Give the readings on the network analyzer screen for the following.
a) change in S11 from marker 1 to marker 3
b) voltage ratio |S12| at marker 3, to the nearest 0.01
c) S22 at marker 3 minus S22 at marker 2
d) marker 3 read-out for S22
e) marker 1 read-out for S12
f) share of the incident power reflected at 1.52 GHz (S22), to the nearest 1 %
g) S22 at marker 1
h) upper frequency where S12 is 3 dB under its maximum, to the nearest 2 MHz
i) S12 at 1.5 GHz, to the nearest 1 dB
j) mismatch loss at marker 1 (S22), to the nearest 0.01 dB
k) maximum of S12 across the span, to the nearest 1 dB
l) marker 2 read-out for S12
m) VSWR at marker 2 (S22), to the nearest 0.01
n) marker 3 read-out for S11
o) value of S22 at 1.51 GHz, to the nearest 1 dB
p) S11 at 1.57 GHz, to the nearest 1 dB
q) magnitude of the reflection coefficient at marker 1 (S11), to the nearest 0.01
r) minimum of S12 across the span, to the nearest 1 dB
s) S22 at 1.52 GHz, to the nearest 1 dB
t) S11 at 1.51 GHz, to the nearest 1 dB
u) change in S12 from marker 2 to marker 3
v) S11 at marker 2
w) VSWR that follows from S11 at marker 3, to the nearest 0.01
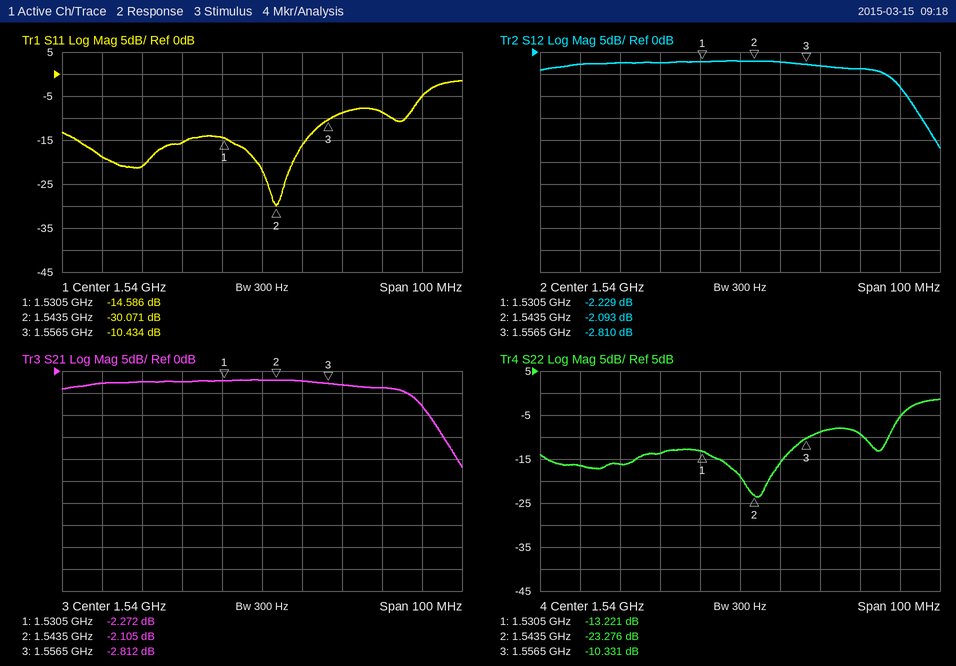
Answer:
4.152 dB
0.72
12.945 dB
-10.331 dB
-2.229 dB
4 %
-13.221 dB
1.576 GHz
-3 dB
0.21 dB
-2 dB
-2.093 dB
1.15
-10.434 dB
-16 dB
-9 dB
0.19
-22 dB
-14 dB
-21 dB
-0.717 dB
-30.071 dB
1.86
